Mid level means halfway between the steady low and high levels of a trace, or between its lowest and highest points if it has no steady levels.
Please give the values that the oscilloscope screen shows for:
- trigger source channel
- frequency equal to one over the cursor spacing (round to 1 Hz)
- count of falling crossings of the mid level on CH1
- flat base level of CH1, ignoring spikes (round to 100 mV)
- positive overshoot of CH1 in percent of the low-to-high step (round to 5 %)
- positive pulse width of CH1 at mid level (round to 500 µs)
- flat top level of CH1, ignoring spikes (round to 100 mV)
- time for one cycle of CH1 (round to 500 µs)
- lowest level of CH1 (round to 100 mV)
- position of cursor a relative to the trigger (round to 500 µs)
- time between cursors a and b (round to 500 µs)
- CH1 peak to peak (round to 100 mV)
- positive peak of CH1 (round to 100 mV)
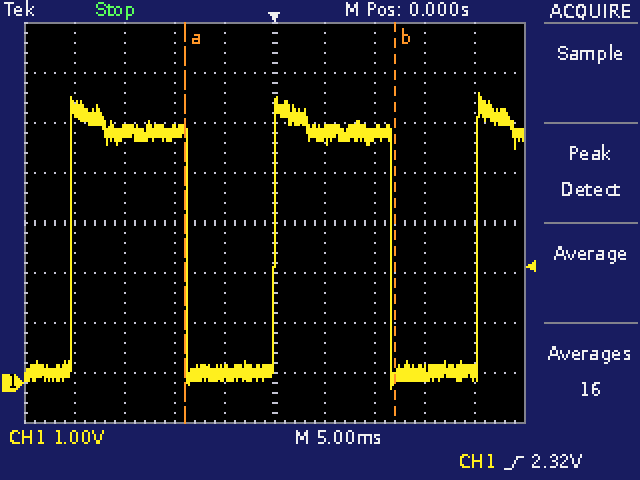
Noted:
CH1
48 Hz
2
200 mV
15 %
11.5 ms
5.0 V
20.5 ms
-100 mV
-9.0 ms
21.0 ms
5.9 V
5.8 V
